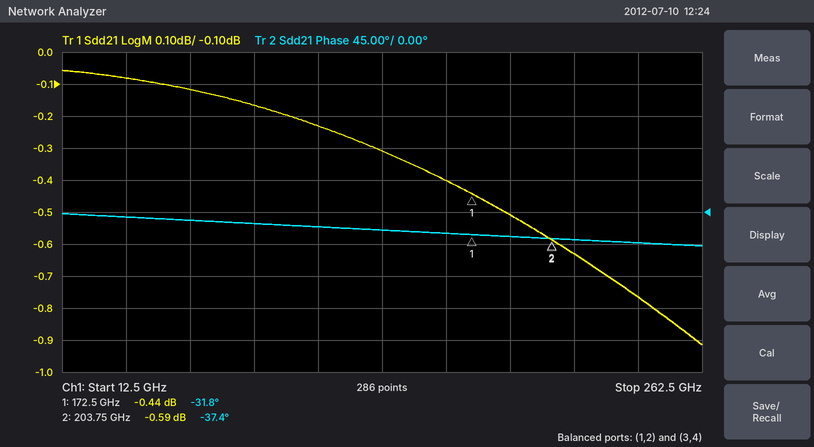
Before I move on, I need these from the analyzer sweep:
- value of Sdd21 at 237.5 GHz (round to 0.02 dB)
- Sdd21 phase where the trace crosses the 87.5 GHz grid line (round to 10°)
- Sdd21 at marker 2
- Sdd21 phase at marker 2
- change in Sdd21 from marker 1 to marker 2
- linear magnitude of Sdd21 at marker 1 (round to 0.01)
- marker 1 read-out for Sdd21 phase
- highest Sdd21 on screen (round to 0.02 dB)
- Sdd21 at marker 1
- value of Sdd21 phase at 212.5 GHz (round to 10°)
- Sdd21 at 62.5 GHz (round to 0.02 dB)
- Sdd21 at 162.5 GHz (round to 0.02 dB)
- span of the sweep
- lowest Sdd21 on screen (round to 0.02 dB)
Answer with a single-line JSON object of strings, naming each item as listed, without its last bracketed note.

{"value of Sdd21 at 237.5 GHz": "-0.76 dB", "Sdd21 phase where the trace crosses the 87.5 GHz grid line": "-20°", "Sdd21 at marker 2": "-0.59 dB", "Sdd21 phase at marker 2": "-37.4°", "change in Sdd21 from marker 1 to marker 2": "-0.15 dB", "linear magnitude of Sdd21 at marker 1": "0.95", "marker 1 read-out for Sdd21 phase": "-31.8°", "highest Sdd21 on screen": "-0.06 dB", "Sdd21 at marker 1": "-0.44 dB", "value of Sdd21 phase at 212.5 GHz": "-40°", "Sdd21 at 62.5 GHz": "-0.12 dB", "Sdd21 at 162.5 GHz": "-0.40 dB", "span of the sweep": "250 GHz", "lowest Sdd21 on screen": "-0.92 dB"}
